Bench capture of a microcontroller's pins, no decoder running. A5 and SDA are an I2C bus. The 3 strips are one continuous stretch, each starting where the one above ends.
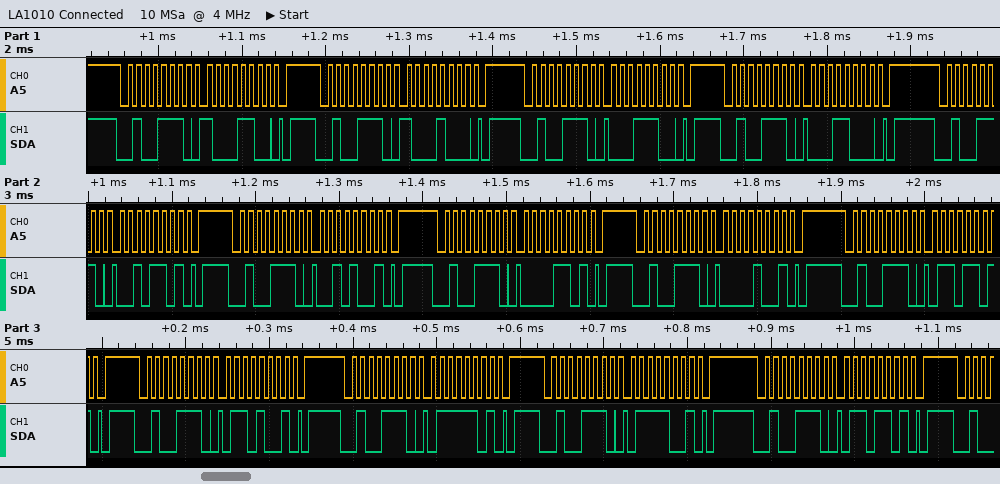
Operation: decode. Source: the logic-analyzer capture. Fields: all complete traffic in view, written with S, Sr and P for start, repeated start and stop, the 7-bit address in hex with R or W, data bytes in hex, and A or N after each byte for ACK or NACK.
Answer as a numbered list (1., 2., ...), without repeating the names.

1. S 27W A 8C A P S 27W A 88 A P S 27W A 1C A P S 27W A 18 A P S 27W A 2D A P S 27W A 29 A P S 27W A 0D A P S 27W A 09 A P S 27W A 6D A P S 27W A 69 A P S 27W A 7D A P S 27W A 79 A P S 27W A 6D A P
